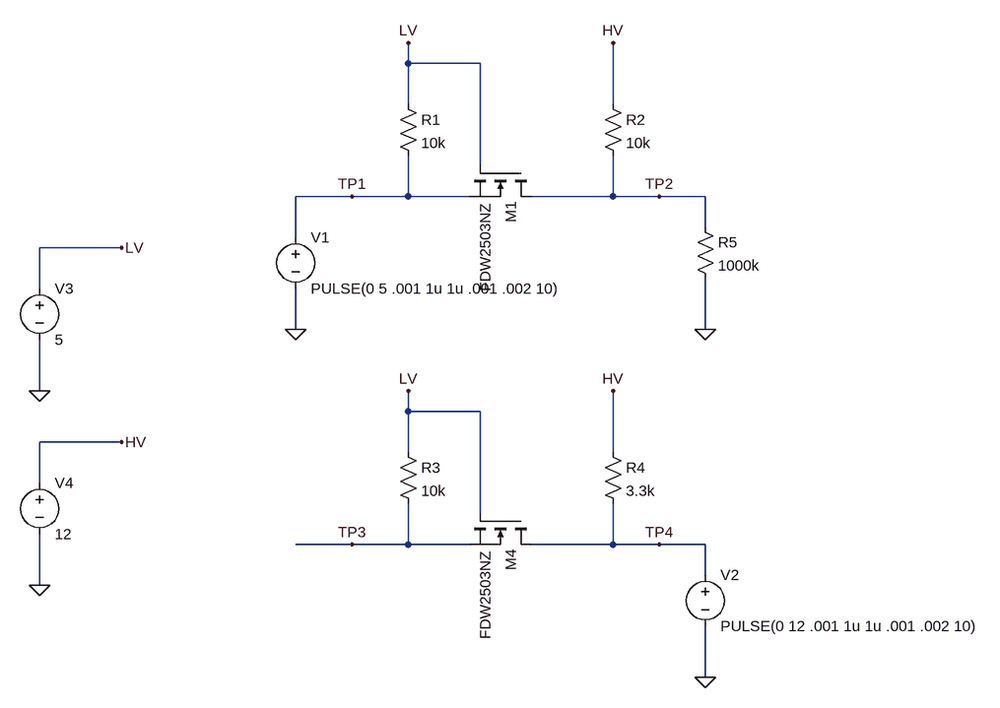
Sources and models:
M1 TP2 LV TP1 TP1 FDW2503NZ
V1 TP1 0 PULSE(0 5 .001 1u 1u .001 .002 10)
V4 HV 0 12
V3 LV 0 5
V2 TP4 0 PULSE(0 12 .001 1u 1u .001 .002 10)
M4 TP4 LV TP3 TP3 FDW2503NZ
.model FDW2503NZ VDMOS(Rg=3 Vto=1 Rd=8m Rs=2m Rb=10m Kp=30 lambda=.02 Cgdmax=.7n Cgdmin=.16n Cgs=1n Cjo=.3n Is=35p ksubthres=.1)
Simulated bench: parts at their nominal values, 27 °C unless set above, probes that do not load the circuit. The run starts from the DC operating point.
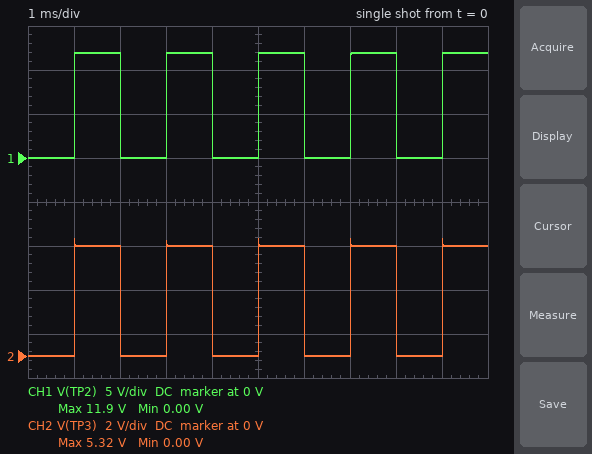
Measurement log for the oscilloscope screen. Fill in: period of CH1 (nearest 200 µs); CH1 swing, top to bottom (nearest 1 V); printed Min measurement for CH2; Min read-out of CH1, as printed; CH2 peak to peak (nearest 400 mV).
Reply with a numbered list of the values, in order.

1. 2.0 ms
2. 12 V
3. 0.00 V
4. 0.00 V
5. 5.2 V
